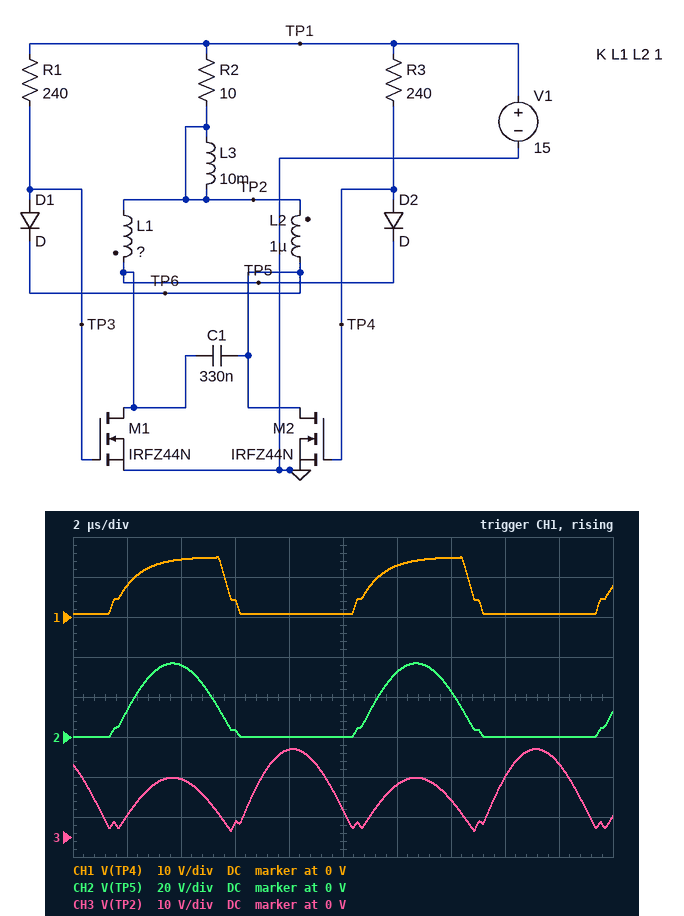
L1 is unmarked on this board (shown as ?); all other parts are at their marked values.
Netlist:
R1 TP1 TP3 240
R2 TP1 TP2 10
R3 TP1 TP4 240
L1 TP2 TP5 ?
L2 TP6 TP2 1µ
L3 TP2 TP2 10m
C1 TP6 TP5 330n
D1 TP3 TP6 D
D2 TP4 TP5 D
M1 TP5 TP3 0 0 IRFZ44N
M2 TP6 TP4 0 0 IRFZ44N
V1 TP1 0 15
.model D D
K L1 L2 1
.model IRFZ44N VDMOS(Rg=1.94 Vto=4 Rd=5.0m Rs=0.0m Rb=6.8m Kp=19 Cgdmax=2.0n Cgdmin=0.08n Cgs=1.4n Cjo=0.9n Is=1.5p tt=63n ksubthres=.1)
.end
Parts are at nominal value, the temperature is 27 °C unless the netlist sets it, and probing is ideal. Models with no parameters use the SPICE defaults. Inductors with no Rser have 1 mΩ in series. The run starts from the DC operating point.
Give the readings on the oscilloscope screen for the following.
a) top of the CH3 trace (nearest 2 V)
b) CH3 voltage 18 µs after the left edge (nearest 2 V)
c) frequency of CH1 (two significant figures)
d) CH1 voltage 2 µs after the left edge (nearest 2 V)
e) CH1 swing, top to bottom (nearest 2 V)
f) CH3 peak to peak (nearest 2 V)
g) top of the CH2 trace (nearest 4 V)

22 V
18 V
110 kHz
8 V
14 V
20 V
36 V
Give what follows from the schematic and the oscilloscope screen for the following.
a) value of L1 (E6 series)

2.2 µH
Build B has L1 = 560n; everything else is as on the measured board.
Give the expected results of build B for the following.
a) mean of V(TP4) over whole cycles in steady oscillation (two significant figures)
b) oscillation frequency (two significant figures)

5.9 V
160 kHz
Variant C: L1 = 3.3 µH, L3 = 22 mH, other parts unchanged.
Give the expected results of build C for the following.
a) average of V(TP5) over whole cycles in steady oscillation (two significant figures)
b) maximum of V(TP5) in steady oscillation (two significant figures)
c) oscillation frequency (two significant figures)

11 V
35 V
98 kHz
